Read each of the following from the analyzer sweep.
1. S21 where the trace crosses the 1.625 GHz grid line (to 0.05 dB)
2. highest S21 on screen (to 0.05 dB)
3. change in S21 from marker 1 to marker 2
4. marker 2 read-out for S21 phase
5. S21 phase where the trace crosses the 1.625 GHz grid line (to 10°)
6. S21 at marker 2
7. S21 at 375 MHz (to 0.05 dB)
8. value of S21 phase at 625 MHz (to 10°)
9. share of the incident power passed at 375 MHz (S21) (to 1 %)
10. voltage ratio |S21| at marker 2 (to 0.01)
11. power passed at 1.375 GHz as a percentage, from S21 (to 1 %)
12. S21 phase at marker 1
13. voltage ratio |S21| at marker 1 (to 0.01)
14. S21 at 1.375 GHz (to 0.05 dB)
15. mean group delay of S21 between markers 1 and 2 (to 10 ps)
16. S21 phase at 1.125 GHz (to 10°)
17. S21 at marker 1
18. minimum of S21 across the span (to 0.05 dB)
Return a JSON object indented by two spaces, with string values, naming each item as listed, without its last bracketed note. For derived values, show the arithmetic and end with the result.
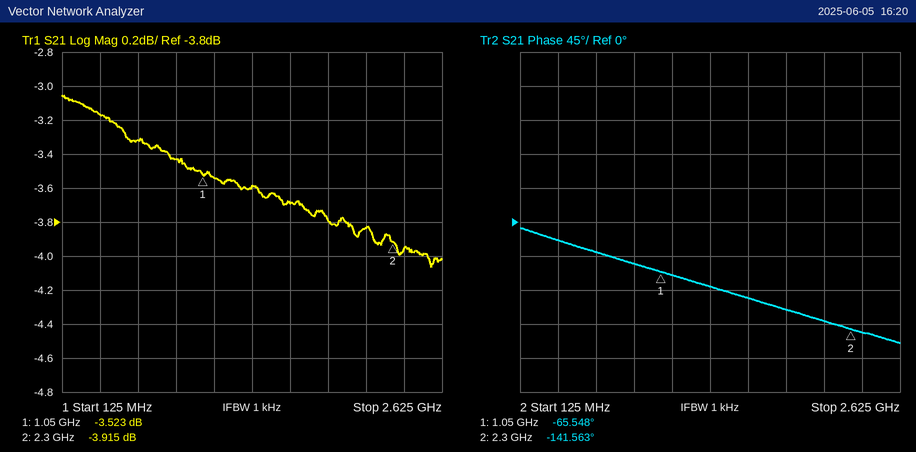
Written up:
{
  "S21 where the trace crosses the 1.625 GHz grid line": "-3.70 dB",
  "highest S21 on screen": "-3.05 dB",
  "change in S21 from marker 1 to marker 2": "-3.915 − (-3.523) = -0.392 dB",
  "marker 2 read-out for S21 phase": "-141.563°",
  "S21 phase where the trace crosses the 1.625 GHz grid line": "-100°",
  "S21 at marker 2": "-3.915 dB",
  "S21 at 375 MHz": "-3.15 dB",
  "value of S21 phase at 625 MHz": "-40°",
  "share of the incident power passed at 375 MHz (S21)": "10^(-3.15/10) ≈ 48 %",
  "voltage ratio |S21| at marker 2": "10^(-3.915/20) ≈ 0.64",
  "power passed at 1.375 GHz as a percentage, from S21": "10^(-3.6/10) ≈ 44 %",
  "S21 phase at marker 1": "-65.548°",
  "voltage ratio |S21| at marker 1": "10^(-3.523/20) ≈ 0.67",
  "S21 at 1.375 GHz": "-3.60 dB",
  "mean group delay of S21 between markers 1 and 2": "−(-141.563° − (-65.548°))/(360° × 1.25 GHz) ≈ 169 ps, so 170 ps to the nearest 10 ps",
  "S21 phase at 1.125 GHz": "-70°",
  "S21 at marker 1": "-3.523 dB",
  "minimum of S21 across the span": "-4.05 dB"
}
